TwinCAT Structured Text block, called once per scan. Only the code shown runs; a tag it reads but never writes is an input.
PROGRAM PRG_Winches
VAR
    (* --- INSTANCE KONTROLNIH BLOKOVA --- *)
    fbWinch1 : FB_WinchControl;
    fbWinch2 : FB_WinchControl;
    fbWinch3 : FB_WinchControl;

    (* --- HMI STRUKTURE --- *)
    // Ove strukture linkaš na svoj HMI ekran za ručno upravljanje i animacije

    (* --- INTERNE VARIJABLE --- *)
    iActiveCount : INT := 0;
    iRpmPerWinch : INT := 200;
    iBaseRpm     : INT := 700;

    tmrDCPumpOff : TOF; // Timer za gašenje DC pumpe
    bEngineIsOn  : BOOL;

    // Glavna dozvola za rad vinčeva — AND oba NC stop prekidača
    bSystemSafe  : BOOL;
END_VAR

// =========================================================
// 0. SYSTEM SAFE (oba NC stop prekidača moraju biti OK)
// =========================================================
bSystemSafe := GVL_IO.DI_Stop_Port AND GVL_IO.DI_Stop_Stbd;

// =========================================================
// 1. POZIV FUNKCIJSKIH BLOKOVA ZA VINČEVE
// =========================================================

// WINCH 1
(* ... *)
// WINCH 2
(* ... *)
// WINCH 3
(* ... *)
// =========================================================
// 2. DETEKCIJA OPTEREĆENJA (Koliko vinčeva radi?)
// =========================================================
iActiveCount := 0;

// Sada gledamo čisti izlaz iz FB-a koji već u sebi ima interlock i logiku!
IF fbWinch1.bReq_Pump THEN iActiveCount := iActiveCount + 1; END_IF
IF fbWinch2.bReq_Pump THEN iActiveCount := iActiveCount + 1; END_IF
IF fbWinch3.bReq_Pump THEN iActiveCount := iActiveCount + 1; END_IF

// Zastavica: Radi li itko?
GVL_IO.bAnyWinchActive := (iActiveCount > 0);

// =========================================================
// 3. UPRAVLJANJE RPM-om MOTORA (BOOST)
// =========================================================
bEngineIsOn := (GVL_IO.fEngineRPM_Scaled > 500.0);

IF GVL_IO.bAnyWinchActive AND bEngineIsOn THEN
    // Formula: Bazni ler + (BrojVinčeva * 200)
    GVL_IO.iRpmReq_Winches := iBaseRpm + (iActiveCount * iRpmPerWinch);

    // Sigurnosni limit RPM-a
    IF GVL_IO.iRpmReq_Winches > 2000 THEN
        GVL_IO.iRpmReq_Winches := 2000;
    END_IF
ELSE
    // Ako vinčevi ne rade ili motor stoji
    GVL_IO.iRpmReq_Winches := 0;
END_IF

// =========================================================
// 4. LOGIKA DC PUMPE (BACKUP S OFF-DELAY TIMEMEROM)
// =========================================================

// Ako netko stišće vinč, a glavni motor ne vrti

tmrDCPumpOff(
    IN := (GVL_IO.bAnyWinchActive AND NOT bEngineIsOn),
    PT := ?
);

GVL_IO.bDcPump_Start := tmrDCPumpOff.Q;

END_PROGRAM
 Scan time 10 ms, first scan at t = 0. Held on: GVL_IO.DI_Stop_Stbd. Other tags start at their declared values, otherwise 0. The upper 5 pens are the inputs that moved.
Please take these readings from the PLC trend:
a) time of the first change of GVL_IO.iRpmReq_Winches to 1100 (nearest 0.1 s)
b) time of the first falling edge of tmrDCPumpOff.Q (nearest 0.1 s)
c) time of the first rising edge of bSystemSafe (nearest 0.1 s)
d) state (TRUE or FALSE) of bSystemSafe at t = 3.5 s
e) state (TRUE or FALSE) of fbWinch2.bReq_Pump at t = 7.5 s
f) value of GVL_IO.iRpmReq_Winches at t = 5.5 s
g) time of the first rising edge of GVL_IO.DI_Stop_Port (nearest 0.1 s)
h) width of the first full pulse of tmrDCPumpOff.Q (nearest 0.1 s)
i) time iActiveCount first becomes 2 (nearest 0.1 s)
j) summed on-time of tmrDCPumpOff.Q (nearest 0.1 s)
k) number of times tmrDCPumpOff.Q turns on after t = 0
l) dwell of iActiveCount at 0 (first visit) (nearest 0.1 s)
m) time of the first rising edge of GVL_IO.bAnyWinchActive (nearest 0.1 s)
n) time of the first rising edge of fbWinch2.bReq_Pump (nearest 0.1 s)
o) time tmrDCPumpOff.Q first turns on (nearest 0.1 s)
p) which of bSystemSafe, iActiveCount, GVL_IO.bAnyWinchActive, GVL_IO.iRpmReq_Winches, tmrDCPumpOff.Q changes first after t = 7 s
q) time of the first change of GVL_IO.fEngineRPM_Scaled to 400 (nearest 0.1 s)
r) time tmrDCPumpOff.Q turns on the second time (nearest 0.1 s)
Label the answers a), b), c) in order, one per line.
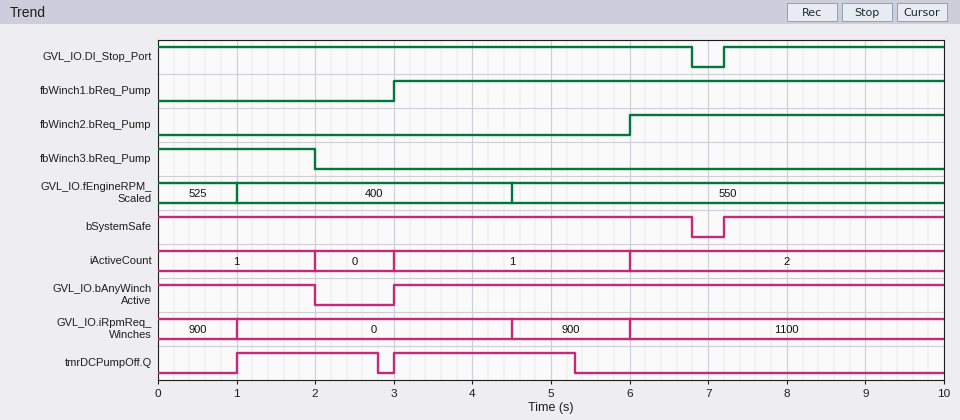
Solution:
a) 6.0 s
b) 2.8 s
c) 7.2 s
d) TRUE
e) TRUE
f) 900
g) 7.2 s
h) 1.8 s
i) 6.0 s
j) 4.1 s
k) 2
l) 1.0 s
m) 3.0 s
n) 6.0 s
o) 1.0 s
p) bSystemSafe
q) 1.0 s
r) 3.0 s
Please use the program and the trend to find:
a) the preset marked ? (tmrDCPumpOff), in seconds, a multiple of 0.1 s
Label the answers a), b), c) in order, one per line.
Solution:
a) 0.8 s
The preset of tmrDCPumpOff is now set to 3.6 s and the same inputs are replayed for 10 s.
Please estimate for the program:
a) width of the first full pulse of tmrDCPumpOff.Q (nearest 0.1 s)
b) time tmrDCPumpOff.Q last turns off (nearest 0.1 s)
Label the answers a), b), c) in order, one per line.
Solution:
a) 7.1 s
b) 8.1 s
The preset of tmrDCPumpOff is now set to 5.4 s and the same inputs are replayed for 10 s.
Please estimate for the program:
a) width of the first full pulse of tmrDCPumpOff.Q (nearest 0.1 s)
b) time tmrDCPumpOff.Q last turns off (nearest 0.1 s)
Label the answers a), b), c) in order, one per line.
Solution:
a) 8.9 s
b) 9.9 s
